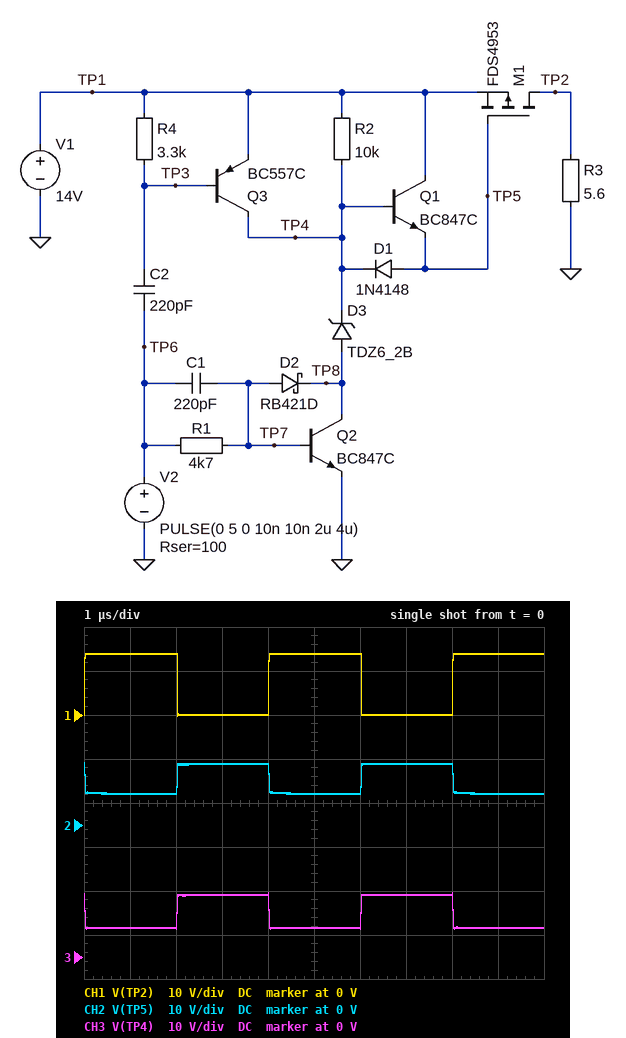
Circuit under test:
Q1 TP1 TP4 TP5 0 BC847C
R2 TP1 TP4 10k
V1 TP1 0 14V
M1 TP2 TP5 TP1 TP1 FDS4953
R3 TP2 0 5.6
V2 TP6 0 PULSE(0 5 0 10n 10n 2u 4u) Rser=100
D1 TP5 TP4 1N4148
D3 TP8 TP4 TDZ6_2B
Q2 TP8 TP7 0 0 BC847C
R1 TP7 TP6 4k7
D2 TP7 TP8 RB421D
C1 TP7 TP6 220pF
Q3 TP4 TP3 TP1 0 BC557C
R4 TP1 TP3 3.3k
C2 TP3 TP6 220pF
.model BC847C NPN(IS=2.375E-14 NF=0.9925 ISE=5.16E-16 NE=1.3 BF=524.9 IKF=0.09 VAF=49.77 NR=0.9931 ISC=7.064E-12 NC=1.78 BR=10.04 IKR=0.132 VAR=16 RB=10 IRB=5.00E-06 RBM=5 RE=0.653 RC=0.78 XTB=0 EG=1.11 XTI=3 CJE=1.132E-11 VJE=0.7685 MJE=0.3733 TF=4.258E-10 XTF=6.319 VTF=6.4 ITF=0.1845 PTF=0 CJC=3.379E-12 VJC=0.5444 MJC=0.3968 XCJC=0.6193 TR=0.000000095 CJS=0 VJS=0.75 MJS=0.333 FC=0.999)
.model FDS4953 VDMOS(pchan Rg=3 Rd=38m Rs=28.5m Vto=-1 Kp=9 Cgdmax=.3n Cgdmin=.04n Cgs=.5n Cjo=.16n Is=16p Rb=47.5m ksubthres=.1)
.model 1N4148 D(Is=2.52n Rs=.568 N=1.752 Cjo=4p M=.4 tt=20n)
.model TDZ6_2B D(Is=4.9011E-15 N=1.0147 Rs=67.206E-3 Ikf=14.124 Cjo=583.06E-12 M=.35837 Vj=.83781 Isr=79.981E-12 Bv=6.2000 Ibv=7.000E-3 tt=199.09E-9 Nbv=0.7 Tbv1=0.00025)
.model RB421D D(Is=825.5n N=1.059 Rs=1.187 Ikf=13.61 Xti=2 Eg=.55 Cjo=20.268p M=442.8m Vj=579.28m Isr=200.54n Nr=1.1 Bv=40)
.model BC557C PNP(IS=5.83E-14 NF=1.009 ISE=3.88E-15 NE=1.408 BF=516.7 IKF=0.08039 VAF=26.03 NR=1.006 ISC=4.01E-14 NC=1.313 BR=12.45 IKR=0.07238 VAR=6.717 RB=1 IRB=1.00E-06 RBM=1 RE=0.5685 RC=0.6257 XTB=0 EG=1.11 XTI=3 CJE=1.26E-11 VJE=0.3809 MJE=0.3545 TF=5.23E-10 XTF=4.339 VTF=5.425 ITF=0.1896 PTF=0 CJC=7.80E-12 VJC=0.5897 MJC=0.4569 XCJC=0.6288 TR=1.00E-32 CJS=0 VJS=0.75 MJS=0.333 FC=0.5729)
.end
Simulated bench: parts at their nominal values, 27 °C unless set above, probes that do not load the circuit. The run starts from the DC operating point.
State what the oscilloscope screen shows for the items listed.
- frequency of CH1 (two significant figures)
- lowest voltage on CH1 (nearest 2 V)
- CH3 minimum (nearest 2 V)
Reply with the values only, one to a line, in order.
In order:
250 kHz
0 V
6 V
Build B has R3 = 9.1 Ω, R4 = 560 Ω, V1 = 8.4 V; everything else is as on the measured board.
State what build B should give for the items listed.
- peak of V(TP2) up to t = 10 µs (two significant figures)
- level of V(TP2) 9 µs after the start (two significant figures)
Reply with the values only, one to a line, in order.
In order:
4.9 V
3.9 V
